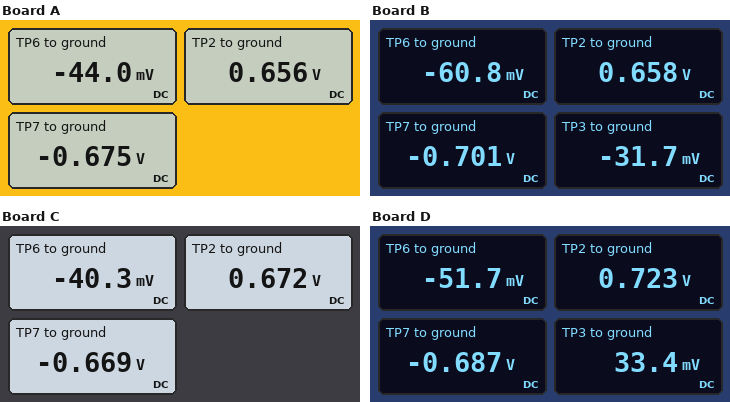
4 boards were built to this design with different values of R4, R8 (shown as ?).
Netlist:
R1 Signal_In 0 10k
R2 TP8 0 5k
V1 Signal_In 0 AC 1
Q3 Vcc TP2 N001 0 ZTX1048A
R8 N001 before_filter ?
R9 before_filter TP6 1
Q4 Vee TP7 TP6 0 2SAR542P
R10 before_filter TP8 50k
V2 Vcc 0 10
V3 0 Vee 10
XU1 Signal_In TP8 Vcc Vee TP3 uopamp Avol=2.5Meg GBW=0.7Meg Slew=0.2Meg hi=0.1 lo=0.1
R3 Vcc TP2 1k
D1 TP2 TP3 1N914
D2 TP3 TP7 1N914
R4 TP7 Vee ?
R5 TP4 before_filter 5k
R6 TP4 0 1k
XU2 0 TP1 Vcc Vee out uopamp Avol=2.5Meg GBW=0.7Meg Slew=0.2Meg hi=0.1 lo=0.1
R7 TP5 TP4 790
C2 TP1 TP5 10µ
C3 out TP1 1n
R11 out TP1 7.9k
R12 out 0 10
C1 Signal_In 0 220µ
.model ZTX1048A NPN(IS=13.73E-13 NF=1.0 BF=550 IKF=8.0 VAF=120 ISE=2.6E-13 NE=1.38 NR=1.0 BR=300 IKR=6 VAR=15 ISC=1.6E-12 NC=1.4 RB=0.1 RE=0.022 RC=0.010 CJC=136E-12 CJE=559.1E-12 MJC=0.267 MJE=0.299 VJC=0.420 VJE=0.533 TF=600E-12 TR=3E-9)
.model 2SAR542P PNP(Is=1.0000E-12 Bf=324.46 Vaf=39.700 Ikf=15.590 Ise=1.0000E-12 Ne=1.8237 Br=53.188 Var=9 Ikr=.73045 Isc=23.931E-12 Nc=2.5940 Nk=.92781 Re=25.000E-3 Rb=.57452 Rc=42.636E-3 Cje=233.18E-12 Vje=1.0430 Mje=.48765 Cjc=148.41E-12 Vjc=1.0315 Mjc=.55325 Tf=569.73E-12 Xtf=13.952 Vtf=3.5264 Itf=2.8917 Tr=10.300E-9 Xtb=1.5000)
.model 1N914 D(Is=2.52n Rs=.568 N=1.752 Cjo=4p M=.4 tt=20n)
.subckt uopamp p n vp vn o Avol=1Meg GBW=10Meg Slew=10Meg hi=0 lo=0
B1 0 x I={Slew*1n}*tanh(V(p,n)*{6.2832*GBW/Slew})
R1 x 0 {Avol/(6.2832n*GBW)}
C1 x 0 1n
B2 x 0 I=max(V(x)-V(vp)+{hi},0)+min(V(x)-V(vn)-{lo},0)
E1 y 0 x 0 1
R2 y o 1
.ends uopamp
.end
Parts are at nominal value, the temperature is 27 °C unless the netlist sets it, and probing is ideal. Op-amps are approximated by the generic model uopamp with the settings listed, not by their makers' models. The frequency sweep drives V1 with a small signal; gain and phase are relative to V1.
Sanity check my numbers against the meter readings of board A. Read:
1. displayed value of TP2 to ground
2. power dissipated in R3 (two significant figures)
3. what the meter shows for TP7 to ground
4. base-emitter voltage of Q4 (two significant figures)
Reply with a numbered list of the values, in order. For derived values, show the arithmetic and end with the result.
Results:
1. 0.656 V
2. (10 V - 656 mV)^2 / 1 kΩ = 87 mW
3. -0.675 V
4. -675 mV - (-44 mV) = -630 mV
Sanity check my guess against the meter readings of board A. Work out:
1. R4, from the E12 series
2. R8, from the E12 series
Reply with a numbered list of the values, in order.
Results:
1. 2.7 kΩ
2. 0.68 Ω
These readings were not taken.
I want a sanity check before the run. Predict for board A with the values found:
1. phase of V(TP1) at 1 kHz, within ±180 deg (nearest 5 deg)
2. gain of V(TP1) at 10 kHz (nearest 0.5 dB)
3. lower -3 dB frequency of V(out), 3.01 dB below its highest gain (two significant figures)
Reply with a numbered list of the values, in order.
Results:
1. 85 deg
2. -18.5 dB
3. 9.8 Hz
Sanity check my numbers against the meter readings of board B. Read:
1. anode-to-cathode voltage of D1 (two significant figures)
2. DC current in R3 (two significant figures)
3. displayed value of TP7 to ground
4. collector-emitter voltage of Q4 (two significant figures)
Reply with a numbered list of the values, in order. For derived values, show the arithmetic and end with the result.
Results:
1. 658 mV - (-31.7 mV) = 690 mV
2. (10 V - 658 mV) / 1 kΩ = 9.3 mA
3. -0.701 V
4. -10 V - (-60.8 mV) = -9.9 V
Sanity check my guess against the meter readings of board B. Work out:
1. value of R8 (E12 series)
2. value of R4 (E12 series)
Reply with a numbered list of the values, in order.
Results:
1. 0.39 Ω
2. 1.5 kΩ
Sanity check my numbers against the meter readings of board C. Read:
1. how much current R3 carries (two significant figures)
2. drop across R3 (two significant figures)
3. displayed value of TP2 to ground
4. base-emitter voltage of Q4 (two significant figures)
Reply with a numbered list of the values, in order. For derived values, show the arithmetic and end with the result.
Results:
1. (10 V - 672 mV) / 1 kΩ = 9.3 mA
2. 10 V - 672 mV = 9.3 V
3. 0.672 V
4. -669 mV - (-40.3 mV) = -630 mV
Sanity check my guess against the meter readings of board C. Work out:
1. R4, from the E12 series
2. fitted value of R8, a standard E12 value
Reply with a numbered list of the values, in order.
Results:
1. 2.2 kΩ
2. 1.2 Ω
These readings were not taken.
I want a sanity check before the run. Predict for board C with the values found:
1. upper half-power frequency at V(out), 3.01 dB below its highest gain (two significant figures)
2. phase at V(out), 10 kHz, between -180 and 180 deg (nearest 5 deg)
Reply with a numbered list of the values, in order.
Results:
1. 16 kHz
2. 140 deg
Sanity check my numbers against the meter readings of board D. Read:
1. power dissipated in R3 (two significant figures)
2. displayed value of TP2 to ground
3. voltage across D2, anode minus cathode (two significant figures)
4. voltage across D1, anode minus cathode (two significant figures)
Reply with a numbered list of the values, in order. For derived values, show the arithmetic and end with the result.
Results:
1. (10 V - 723 mV)^2 / 1 kΩ = 86 mW
2. 0.723 V
3. 33.4 mV - (-687 mV) = 720 mV
4. 723 mV - 33.4 mV = 690 mV
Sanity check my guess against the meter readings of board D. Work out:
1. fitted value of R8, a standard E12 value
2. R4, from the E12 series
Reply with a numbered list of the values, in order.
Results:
1. 1.8 Ω
2. 560 Ω
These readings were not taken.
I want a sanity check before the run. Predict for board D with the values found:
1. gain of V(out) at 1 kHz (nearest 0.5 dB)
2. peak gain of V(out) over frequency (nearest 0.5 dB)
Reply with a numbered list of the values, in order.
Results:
1. 19.0 dB
2. 19.0 dB
